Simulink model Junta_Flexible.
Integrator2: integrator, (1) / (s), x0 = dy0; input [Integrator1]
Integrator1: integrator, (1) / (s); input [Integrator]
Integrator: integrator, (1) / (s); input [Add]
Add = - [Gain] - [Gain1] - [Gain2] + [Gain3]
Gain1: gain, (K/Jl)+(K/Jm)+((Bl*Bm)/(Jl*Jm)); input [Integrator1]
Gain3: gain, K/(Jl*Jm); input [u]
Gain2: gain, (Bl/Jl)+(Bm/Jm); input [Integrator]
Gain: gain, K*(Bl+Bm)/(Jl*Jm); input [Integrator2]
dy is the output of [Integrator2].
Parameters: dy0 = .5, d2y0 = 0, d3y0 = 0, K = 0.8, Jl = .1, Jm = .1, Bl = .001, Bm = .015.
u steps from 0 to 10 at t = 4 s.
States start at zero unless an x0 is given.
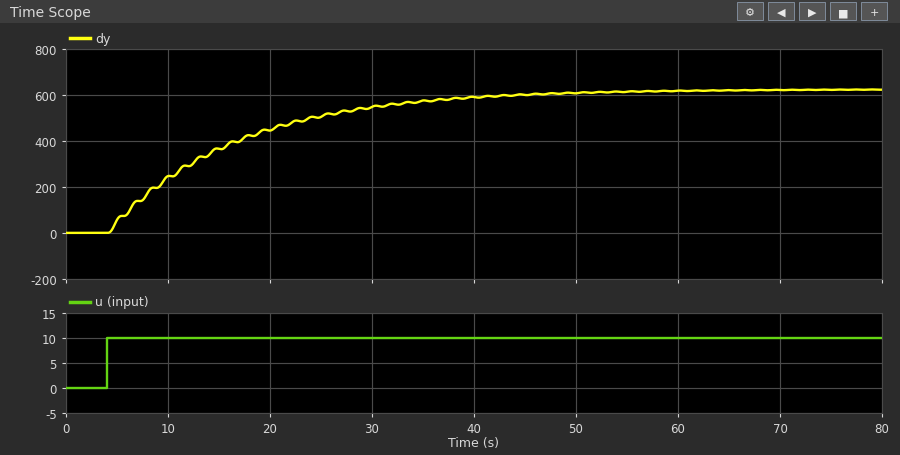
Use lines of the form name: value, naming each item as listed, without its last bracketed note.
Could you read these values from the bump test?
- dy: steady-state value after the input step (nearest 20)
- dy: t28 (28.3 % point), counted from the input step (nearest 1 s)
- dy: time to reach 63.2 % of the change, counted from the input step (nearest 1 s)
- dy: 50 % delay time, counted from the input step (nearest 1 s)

dy: steady-state value after the input step: 620
dy: t28 (28.3 % point), counted from the input step: 4 s
dy: time to reach 63.2 % of the change, counted from the input step: 12 s
dy: 50 % delay time, counted from the input step: 9 s
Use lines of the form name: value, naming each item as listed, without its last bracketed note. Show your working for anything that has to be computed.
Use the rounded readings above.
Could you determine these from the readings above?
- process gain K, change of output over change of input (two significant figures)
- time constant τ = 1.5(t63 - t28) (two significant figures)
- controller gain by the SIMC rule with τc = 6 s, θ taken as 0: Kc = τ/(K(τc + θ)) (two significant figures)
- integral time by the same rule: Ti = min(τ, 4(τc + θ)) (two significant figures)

process gain K, change of output over change of input: (620 - 0) / 10 = 62
time constant τ = 1.5(t63 - t28): 1.5 × (12 - 4) = 12 s
controller gain by the SIMC rule with τc = 6 s, θ taken as 0: Kc = τ/(K(τc + θ)): 12 / (62 × (6 + 0)) = 0.032
integral time by the same rule: Ti = min(τ, 4(τc + θ)): min(12, 4 × (6 + 0)) = 12 s
